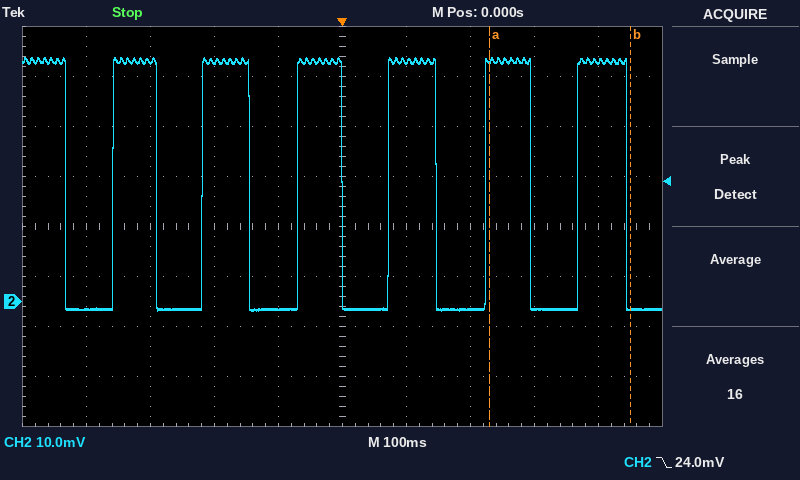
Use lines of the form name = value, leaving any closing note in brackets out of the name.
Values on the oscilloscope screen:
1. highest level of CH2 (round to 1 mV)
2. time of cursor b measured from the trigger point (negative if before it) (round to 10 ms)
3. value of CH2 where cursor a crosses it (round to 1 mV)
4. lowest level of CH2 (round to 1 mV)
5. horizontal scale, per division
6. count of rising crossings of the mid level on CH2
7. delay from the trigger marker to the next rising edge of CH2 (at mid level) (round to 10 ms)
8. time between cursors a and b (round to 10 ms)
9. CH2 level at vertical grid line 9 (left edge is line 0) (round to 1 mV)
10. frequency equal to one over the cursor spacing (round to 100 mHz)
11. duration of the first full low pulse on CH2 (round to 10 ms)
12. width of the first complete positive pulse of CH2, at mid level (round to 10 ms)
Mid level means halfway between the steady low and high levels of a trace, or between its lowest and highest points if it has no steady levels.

highest level of CH2 = 49 mV
time of cursor b measured from the trigger point (negative if before it) = +450 ms
value of CH2 where cursor a crosses it = 48 mV
lowest level of CH2 = -2 mV
horizontal scale, per division = 100 ms
count of rising crossings of the mid level on CH2 = 6
delay from the trigger marker to the next rising edge of CH2 (at mid level) = 70 ms
time between cursors a and b = 220 ms
CH2 level at vertical grid line 9 (left edge is line 0) = 48 mV
frequency equal to one over the cursor spacing = 4.5 Hz
duration of the first full low pulse on CH2 = 70 ms
width of the first complete positive pulse of CH2, at mid level = 70 ms
